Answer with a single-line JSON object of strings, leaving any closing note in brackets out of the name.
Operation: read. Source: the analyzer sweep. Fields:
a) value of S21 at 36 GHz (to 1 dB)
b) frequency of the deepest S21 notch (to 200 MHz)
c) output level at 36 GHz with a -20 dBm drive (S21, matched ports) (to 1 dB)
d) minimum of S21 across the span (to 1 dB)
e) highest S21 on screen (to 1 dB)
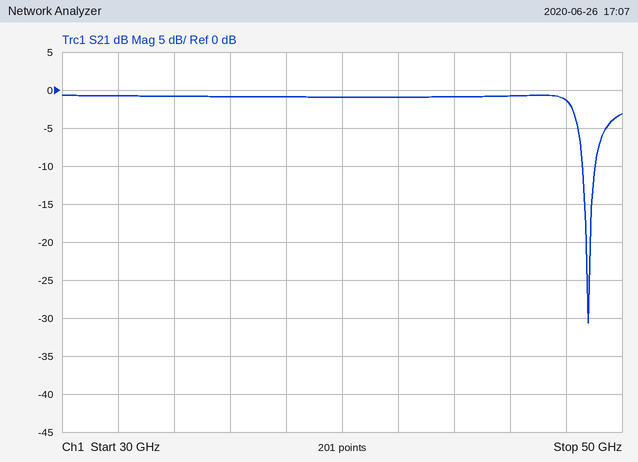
{"value of S21 at 36 GHz": "-1 dB", "frequency of the deepest S21 notch": "48.8 GHz", "output level at 36 GHz with a -20 dBm drive (S21, matched ports)": "-21 dBm", "minimum of S21 across the span": "-31 dB", "highest S21 on screen": "-1 dB"}
